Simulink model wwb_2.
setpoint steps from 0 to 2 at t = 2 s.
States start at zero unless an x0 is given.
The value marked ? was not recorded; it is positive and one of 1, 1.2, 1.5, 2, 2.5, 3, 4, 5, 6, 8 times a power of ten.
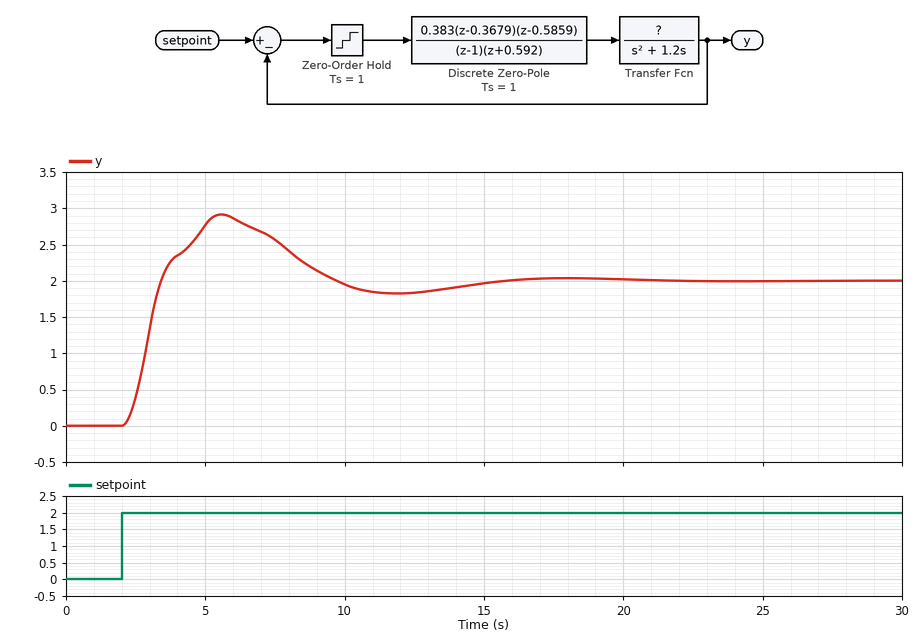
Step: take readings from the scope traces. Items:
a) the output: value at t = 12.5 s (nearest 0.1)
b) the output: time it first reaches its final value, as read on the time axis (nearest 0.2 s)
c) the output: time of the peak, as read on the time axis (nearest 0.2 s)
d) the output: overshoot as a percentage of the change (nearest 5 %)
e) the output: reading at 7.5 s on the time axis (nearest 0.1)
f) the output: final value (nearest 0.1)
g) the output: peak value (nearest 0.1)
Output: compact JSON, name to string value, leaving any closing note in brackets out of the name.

{"the output: value at t = 12.5 s": "1.8", "the output: time it first reaches its final value, as read on the time axis": "3.4 s", "the output: time of the peak, as read on the time axis": "5.6 s", "the output: overshoot as a percentage of the change": "45 %", "the output: reading at 7.5 s on the time axis": "2.6", "the output: final value": "2.0", "the output: peak value": "2.9"}
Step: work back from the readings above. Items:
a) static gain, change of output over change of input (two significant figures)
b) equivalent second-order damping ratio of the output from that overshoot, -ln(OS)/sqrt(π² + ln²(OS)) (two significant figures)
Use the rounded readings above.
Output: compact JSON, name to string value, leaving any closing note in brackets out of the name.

{"static gain, change of output over change of input": "1.0", "equivalent second-order damping ratio of the output from that overshoot, -ln(OS)/sqrt(π² + ln²(OS))": "0.25"}
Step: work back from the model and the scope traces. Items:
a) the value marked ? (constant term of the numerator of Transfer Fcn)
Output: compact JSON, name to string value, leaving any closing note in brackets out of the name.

{"the value marked ?": "5"}
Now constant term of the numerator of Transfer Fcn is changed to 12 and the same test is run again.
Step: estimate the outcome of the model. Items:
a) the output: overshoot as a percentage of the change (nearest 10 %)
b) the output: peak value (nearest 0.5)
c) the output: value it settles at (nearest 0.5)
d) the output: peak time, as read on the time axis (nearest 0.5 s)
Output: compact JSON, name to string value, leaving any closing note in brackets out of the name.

{"the output: overshoot as a percentage of the change": "110 %", "the output: peak value": "4.0", "the output: value it settles at": "2.0", "the output: peak time, as read on the time axis": "3.5 s"}
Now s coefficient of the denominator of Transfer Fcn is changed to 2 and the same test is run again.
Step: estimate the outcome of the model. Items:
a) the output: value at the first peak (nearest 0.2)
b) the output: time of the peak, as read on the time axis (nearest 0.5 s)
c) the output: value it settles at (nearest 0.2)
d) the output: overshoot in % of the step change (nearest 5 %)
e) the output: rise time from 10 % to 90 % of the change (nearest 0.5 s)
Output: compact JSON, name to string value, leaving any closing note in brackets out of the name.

{"the output: value at the first peak": "2.8", "the output: time of the peak, as read on the time axis": "7.5 s", "the output: value it settles at": "2.0", "the output: overshoot in % of the step change": "40 %", "the output: rise time from 10 % to 90 % of the change": "2.0 s"}
